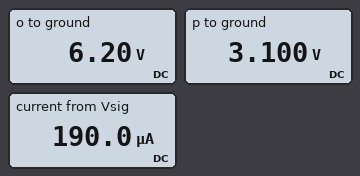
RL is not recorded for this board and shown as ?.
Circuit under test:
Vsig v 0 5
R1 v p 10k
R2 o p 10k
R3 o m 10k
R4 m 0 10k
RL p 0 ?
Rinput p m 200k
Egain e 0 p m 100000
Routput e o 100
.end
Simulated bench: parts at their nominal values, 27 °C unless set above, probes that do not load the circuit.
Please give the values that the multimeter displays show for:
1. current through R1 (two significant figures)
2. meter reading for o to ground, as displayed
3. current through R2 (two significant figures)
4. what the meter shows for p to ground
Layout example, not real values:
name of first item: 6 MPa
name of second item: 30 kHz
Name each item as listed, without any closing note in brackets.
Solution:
current through R1: 190 µA
meter reading for o to ground, as displayed: 6.20 V
current through R2: 310 µA
what the meter shows for p to ground: 3.100 V
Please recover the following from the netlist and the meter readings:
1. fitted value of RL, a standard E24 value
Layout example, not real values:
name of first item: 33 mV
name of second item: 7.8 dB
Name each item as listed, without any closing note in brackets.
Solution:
fitted value of RL, a standard E24 value: 6.2 kΩ
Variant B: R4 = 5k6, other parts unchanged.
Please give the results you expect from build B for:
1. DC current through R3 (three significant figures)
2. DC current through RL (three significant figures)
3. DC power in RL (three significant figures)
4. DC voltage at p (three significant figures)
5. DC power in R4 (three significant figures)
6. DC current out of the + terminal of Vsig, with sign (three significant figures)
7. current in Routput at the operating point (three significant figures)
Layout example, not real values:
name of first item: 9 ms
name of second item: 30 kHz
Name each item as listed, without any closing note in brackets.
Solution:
DC current through R3: 1.08 mA
DC current through RL: 975 µA
DC power in RL: 5.89 mW
DC voltage at p: 6.04 V
DC power in R4: 6.52 mW
DC current out of the + terminal of Vsig, with sign: -104 µA
current in Routput at the operating point: 2.16 mA
